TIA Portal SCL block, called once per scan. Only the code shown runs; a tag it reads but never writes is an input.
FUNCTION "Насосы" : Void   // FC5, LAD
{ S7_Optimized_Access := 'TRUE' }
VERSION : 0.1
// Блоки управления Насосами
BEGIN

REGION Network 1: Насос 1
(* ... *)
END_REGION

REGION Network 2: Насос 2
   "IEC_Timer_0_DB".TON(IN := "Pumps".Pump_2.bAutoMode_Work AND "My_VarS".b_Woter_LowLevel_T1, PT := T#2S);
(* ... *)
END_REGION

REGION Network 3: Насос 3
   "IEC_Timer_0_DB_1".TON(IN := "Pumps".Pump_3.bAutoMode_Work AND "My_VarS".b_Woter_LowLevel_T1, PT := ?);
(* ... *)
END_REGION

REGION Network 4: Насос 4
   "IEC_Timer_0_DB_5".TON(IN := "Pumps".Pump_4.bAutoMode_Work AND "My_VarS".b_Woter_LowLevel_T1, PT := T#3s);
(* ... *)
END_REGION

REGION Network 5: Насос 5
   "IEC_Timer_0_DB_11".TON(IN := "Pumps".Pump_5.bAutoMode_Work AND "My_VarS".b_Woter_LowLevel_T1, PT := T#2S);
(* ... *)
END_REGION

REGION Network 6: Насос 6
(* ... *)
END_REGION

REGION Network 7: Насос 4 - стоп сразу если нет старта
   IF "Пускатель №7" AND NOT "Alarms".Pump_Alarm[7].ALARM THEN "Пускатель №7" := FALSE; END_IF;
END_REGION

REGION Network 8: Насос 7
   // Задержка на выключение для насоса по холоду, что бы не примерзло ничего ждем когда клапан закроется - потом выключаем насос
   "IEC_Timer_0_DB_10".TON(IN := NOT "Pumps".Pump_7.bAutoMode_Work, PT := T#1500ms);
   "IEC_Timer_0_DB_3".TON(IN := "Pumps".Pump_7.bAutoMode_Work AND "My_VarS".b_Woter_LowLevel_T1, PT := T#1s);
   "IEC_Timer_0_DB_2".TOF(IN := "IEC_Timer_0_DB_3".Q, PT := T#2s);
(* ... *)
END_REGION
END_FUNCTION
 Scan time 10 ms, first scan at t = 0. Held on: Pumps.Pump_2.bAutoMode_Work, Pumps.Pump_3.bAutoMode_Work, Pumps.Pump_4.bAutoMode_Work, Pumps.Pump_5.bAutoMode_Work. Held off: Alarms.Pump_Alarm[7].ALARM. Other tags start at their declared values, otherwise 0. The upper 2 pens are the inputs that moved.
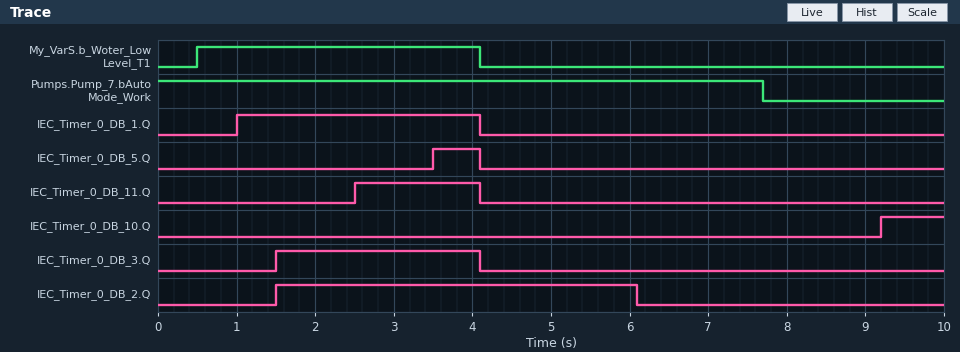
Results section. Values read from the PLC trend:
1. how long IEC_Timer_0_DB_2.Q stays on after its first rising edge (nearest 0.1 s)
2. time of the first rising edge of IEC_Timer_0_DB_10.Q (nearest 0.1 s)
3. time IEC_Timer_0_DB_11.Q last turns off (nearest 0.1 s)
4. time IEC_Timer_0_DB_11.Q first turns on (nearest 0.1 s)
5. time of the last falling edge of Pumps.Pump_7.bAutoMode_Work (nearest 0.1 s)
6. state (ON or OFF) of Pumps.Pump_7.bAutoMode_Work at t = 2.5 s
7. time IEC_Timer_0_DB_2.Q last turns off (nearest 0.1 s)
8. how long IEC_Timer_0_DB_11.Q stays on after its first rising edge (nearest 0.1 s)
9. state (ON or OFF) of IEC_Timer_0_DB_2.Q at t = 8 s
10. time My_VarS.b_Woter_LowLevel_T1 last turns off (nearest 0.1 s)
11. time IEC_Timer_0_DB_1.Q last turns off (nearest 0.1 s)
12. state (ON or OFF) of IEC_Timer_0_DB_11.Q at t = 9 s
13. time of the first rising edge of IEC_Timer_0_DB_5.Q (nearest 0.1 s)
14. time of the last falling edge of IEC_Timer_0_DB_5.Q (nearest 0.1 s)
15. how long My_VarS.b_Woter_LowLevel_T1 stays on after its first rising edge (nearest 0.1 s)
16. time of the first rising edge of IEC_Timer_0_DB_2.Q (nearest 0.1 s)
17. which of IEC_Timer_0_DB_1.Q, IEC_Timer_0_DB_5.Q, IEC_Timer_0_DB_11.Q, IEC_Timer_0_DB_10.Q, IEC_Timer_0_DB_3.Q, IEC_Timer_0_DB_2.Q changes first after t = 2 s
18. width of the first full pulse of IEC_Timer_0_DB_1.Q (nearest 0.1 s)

4.6 s
9.2 s
4.1 s
2.5 s
7.7 s
ON
6.1 s
1.6 s
OFF
4.1 s
4.1 s
OFF
3.5 s
4.1 s
3.6 s
1.5 s
IEC_Timer_0_DB_11.Q
3.1 s
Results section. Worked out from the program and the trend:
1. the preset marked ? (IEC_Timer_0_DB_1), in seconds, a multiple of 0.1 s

0.5 s
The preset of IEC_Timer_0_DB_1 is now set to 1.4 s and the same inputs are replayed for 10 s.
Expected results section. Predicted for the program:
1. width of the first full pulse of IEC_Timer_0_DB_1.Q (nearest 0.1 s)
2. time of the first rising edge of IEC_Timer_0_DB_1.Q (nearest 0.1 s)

2.2 s
1.9 s
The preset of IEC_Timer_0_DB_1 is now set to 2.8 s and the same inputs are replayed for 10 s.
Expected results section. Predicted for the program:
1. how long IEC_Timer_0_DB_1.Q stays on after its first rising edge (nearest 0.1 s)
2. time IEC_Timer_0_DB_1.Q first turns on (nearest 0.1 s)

0.8 s
3.3 s
